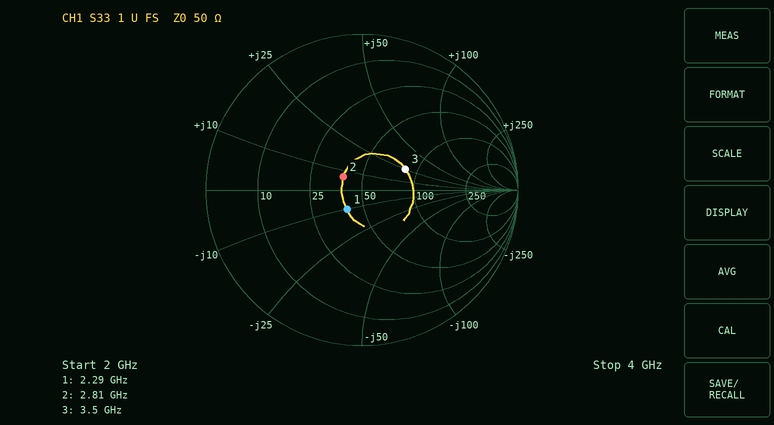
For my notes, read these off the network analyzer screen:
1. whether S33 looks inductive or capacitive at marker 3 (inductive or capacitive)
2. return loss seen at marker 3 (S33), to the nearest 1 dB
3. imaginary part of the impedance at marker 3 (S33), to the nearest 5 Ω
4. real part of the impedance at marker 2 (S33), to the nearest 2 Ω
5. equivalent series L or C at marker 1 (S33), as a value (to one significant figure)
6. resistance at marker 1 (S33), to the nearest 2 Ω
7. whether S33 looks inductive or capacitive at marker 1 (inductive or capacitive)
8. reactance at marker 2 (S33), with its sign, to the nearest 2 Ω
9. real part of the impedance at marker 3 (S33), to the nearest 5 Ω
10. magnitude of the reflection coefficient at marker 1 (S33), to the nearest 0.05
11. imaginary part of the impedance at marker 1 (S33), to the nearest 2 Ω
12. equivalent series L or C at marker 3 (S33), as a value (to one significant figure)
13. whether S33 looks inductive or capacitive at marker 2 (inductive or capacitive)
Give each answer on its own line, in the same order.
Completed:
inductive
10 dB
+25 Ω
38 Ω
7 pF
40 Ω
capacitive
+6 Ω
85 Ω
0.15
-10 Ω
1 nH
inductive
